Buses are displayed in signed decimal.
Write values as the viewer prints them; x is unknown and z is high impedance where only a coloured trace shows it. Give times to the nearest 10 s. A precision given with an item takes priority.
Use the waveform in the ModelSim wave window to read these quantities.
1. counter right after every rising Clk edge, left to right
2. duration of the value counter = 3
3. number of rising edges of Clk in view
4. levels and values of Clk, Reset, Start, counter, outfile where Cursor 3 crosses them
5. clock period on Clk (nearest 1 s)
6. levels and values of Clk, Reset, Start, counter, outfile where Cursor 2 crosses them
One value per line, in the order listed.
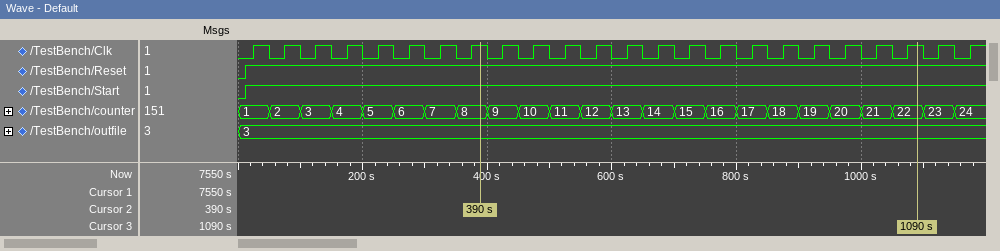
1, 2, 3, 4, 5, 6, 7, 8, 9, 10, 11, 12, 13, 14, 15, 16, 17, 18, 19, 20, 21, 22, 23, 24
50 s
24
Clk=1, Reset=1, Start=1, counter=22, outfile=3
50 s
Clk=1, Reset=1, Start=1, counter=8, outfile=3
